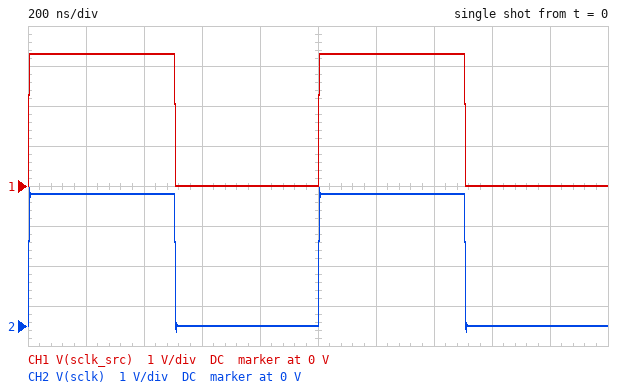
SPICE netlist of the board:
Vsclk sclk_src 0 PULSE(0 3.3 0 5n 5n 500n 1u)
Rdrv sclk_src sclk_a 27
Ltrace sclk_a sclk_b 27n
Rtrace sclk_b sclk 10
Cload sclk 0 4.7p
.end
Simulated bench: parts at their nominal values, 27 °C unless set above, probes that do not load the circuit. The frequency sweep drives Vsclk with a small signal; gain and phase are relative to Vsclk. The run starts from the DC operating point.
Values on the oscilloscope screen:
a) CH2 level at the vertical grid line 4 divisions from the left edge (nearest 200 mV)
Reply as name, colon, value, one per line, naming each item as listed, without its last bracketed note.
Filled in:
CH2 level at the vertical grid line 4 divisions from the left edge: 0 V
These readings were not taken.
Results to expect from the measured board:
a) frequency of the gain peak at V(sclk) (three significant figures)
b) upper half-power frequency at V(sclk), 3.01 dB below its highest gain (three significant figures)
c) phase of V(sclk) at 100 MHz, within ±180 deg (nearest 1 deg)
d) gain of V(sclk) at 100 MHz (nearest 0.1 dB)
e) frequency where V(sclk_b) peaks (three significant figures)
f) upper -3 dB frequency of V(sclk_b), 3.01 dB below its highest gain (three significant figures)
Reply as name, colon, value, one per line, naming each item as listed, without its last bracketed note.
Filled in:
frequency of the gain peak at V(sclk): 419 MHz
upper half-power frequency at V(sclk), 3.01 dB below its highest gain: 520 MHz
phase of V(sclk) at 100 MHz, within ±180 deg: -7 deg
gain of V(sclk) at 100 MHz: 0.4 dB
frequency where V(sclk_b) peaks: 420 MHz
upper -3 dB frequency of V(sclk_b), 3.01 dB below its highest gain: 521 MHz
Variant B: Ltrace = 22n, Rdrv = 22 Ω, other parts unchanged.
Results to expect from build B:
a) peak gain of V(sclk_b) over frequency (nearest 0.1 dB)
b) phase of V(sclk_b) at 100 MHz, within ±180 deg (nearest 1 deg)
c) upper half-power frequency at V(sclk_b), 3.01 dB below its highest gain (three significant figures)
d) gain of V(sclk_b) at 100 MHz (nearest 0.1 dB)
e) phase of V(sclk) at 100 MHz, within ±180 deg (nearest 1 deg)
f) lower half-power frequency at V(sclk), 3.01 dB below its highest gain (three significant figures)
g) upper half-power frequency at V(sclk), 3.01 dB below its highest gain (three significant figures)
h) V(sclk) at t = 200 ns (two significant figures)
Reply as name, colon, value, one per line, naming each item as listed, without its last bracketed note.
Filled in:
peak gain of V(sclk_b) over frequency: 6.9 dB
phase of V(sclk_b) at 100 MHz, within ±180 deg: -4 deg
upper half-power frequency at V(sclk_b), 3.01 dB below its highest gain: 575 MHz
gain of V(sclk_b) at 100 MHz: 0.3 dB
phase of V(sclk) at 100 MHz, within ±180 deg: -6 deg
lower half-power frequency at V(sclk), 3.01 dB below its highest gain: 327 MHz
upper half-power frequency at V(sclk), 3.01 dB below its highest gain: 574 MHz
V(sclk) at t = 200 ns: 3.3 V
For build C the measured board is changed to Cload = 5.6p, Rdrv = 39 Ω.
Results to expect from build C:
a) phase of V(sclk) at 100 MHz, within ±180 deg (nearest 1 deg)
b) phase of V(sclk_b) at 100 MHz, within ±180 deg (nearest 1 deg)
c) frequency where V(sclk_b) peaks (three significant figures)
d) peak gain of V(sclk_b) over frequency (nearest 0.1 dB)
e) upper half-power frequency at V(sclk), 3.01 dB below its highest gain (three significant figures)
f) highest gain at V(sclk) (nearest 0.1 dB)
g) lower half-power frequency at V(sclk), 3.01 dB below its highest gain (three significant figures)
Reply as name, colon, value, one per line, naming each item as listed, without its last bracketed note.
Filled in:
phase of V(sclk) at 100 MHz, within ±180 deg: -10 deg
phase of V(sclk_b) at 100 MHz, within ±180 deg: -8 deg
frequency where V(sclk_b) peaks: 356 MHz
peak gain of V(sclk_b) over frequency: 3.7 dB
upper half-power frequency at V(sclk), 3.01 dB below its highest gain: 486 MHz
highest gain at V(sclk): 3.6 dB
lower half-power frequency at V(sclk), 3.01 dB below its highest gain: 123 MHz
